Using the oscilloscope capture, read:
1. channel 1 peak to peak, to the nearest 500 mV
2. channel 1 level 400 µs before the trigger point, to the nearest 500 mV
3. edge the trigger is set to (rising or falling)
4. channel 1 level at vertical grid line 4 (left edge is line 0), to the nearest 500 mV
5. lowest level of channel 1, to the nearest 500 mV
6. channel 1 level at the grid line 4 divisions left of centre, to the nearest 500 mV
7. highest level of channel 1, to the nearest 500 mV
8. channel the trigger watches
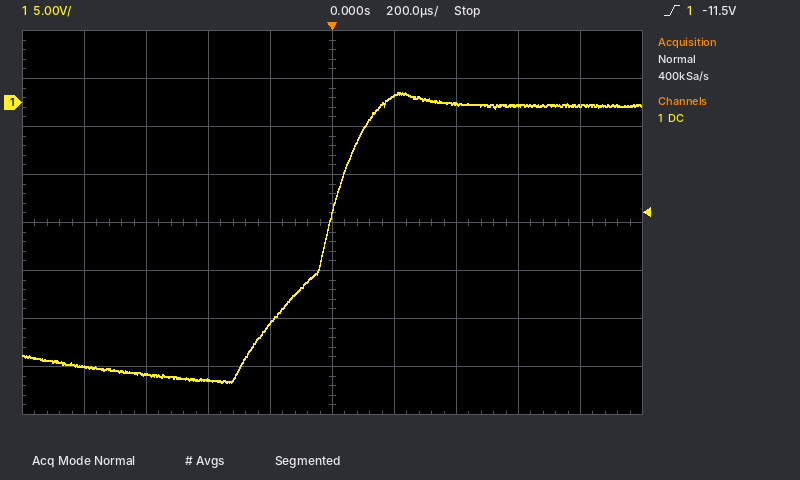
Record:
30.0 V
-29.0 V
rising
-23.0 V
-29.0 V
-27.5 V
1.0 V
channel 1
